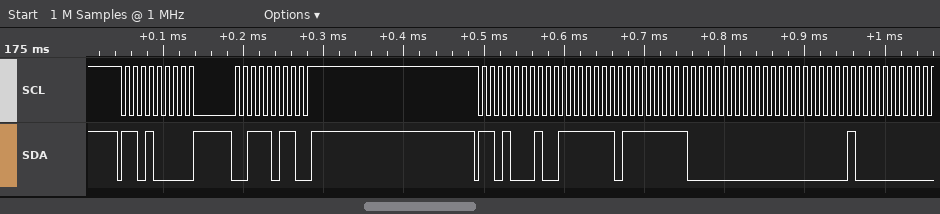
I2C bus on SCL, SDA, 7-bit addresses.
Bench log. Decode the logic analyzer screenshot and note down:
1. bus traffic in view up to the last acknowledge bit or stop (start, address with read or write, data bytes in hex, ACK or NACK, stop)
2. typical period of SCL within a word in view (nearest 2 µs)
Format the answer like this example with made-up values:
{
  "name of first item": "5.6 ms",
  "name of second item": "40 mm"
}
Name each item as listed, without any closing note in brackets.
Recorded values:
{
  "bus traffic in view up to the last acknowledge bit or stop": "start, address 68 write ACK, 3B ACK, stop, start, address 68 read ACK, 7F ACK, FF ACK, 00 ACK, 00 ACK, 40 ACK",
  "typical period of SCL within a word in view": "10 µs"
}
